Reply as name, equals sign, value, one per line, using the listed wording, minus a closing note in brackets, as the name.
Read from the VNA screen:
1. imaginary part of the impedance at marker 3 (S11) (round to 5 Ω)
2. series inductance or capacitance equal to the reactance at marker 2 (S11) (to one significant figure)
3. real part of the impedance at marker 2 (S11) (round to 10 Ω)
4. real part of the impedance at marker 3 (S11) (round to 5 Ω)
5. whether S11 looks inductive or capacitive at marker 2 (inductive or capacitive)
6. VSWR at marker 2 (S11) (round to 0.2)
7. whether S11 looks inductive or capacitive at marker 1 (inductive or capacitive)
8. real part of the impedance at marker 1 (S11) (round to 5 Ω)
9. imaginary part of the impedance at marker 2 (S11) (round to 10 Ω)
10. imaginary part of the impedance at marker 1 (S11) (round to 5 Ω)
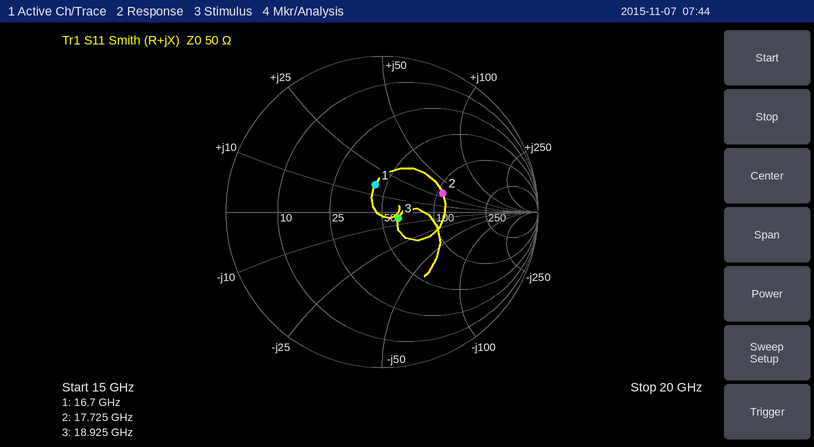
imaginary part of the impedance at marker 3 (S11) = -5 Ω
series inductance or capacitance equal to the reactance at marker 2 (S11) = 300 pH
real part of the impedance at marker 2 (S11) = 110 Ω
real part of the impedance at marker 3 (S11) = 60 Ω
whether S11 looks inductive or capacitive at marker 2 = inductive
VSWR at marker 2 (S11) = 2.4
whether S11 looks inductive or capacitive at marker 1 = inductive
real part of the impedance at marker 1 (S11) = 45 Ω
imaginary part of the impedance at marker 2 (S11) = +30 Ω
imaginary part of the impedance at marker 1 (S11) = +15 Ω
